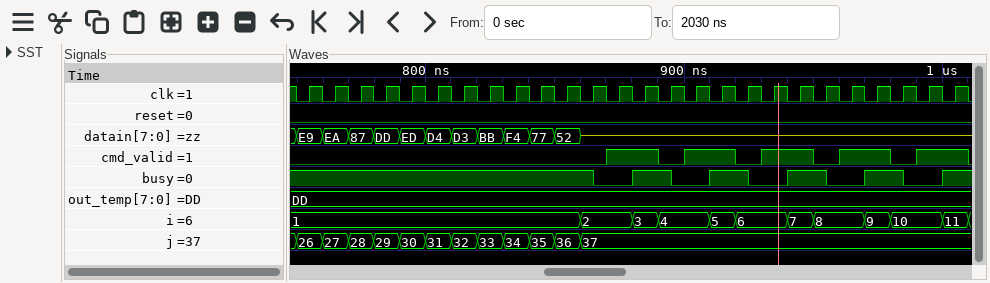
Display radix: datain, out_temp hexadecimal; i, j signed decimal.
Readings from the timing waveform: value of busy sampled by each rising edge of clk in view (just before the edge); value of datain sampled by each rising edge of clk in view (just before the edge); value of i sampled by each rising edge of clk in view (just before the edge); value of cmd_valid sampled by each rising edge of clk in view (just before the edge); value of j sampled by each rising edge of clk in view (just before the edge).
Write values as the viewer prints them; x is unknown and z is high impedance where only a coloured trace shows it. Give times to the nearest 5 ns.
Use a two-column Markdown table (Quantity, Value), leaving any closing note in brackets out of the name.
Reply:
| Quantity | Value |
|---|---|
| value of busy sampled by each rising edge of clk in view | 1 1 1 1 1 1 1 1 1 1 1 1 0 1 1 0 1 1 0 1 1 0 1 1 0 1 |
| value of datain sampled by each rising edge of clk in view | E9, EA, 87, DD, ED, D4, D3, BB, F4, 77, 52, z, z, z, z, z, z, z, z, z, z, z, z, z, z, z |
| value of i sampled by each rising edge of clk in view | 1, 1, 1, 1, 1, 1, 1, 1, 1, 1, 1, 2, 2, 3, 4, 4, 5, 6, 6, 7, 8, 8, 9, 10, 10, 11 |
| value of cmd_valid sampled by each rising edge of clk in view | 0 0 0 0 0 0 0 0 0 0 0 0 1 1 0 1 1 0 1 1 0 1 1 0 1 1 |
| value of j sampled by each rising edge of clk in view | 26, 27, 28, 29, 30, 31, 32, 33, 34, 35, 36, 37, 37, 37, 37, 37, 37, 37, 37, 37, 37, 37, 37, 37, 37, 37 |
